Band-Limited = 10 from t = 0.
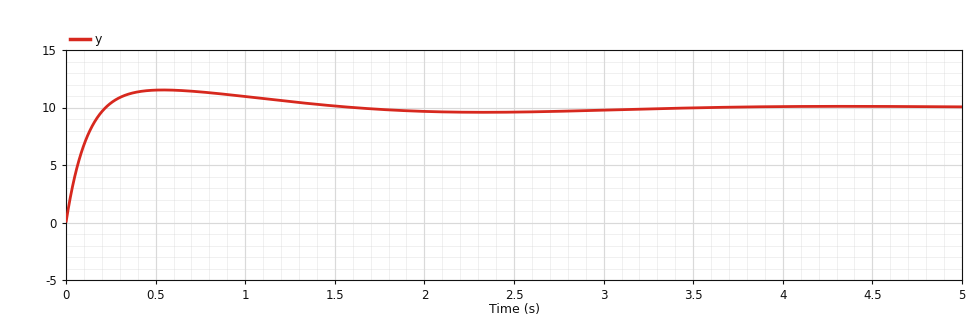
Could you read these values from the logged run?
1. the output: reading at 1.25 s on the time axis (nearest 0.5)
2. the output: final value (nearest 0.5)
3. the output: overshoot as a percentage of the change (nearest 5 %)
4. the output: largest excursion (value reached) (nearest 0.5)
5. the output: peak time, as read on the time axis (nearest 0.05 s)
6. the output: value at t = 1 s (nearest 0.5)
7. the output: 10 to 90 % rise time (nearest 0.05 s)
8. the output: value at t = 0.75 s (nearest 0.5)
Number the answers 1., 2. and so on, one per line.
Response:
1. 10.5
2. 10.0
3. 15 %
4. 11.5
5. 0.55 s
6. 11.0
7. 0.15 s
8. 11.5
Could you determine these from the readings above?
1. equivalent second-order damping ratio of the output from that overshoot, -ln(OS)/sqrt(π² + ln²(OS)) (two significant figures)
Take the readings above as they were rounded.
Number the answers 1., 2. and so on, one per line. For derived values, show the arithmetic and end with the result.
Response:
1. ln(0.15) = -1.897; 1.897 / sqrt(9.870 + 3.599) = 0.52
